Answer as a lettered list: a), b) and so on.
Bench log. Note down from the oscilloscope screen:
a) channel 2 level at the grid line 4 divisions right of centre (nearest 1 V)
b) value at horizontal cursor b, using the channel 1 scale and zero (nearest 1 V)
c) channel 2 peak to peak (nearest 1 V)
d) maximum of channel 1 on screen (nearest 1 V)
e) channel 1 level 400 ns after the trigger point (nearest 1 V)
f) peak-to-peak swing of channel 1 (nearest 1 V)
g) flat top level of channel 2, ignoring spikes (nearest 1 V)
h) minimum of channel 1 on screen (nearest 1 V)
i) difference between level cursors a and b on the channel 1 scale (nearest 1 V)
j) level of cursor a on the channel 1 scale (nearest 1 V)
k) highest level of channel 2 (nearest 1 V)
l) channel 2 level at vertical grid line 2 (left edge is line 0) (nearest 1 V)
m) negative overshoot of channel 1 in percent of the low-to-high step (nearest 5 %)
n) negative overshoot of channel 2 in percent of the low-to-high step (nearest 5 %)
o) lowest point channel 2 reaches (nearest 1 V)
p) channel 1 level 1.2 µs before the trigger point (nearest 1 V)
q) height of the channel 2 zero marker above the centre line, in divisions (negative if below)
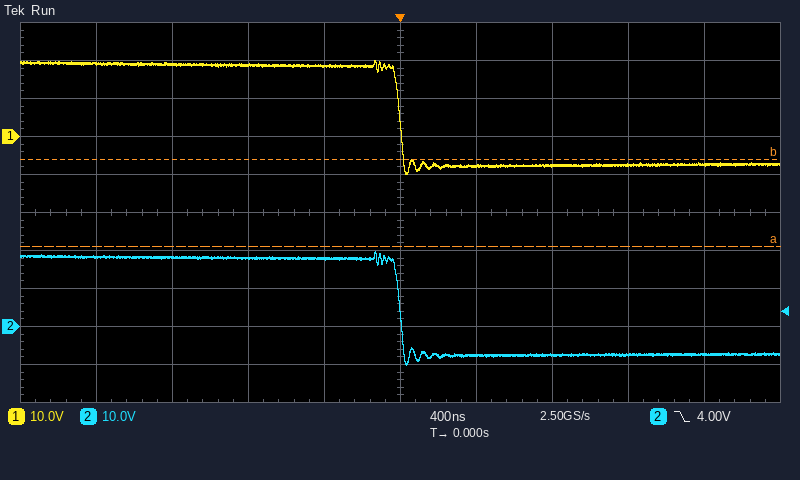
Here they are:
a) -7 V
b) -6 V
c) 30 V
d) 20 V
e) -8 V
f) 30 V
g) 18 V
h) -10 V
i) 23 V
j) -29 V
k) 20 V
l) 18 V
m) 10 %
n) 10 %
o) -10 V
p) 19 V
q) -3.0 div
